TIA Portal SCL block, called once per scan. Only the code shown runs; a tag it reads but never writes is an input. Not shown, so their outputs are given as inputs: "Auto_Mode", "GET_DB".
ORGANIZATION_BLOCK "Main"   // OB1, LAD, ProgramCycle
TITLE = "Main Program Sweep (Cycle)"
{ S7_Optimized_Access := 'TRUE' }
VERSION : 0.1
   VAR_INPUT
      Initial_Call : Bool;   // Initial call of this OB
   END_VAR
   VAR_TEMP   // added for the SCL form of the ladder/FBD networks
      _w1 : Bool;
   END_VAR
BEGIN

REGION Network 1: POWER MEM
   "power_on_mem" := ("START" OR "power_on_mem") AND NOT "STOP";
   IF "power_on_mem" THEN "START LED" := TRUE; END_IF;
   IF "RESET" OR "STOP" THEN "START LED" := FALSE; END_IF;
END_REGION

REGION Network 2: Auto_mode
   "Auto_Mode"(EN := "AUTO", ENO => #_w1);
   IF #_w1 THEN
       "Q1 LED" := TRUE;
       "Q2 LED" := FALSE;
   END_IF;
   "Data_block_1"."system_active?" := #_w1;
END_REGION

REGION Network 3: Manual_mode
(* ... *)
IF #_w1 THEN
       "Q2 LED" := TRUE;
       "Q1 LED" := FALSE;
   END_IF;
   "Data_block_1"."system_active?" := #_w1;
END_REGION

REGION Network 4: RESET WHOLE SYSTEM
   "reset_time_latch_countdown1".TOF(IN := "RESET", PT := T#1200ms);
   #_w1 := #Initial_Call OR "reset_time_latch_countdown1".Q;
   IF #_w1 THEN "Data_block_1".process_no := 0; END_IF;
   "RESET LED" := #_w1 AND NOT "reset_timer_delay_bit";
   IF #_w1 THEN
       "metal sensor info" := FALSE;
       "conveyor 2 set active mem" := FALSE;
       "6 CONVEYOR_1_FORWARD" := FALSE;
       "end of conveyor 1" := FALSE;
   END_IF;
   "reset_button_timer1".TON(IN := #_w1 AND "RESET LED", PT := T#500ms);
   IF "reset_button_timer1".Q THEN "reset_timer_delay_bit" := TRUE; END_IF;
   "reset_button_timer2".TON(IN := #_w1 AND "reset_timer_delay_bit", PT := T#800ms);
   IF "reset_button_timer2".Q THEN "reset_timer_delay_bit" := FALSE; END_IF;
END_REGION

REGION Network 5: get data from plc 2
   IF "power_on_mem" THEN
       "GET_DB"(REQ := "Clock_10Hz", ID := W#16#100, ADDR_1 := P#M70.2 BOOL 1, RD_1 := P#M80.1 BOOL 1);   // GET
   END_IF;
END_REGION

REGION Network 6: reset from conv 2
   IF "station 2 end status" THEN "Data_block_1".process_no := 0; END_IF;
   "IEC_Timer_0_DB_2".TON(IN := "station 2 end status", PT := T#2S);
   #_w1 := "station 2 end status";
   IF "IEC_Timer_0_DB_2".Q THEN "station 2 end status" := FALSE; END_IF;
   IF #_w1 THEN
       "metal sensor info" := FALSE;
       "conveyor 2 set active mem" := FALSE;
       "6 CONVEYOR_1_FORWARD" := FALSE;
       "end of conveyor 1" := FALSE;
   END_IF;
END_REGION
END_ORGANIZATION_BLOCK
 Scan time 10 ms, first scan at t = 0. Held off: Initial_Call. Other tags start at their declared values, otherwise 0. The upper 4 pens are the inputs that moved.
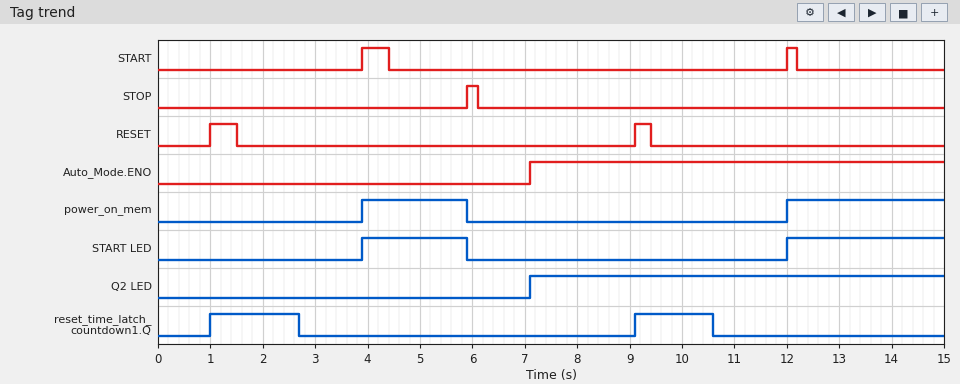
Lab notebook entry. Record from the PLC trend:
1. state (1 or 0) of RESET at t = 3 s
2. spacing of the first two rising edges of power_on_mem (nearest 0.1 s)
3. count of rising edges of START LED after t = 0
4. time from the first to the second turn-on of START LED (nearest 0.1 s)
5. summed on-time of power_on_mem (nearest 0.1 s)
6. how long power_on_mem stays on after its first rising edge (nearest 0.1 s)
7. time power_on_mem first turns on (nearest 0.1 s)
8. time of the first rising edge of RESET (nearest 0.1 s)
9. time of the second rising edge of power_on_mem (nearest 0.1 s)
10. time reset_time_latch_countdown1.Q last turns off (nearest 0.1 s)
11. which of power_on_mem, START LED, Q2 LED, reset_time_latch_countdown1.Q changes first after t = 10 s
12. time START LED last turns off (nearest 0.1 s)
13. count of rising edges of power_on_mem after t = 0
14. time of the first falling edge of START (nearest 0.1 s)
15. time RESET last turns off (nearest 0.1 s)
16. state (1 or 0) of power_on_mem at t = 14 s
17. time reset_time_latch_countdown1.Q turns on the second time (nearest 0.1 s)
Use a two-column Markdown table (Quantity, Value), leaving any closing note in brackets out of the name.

| Quantity | Value |
|---|---|
| state (1 or 0) of RESET at t = 3 s | 0 |
| spacing of the first two rising edges of power_on_mem | 8.1 s |
| count of rising edges of START LED after t = 0 | 2 |
| time from the first to the second turn-on of START LED | 8.1 s |
| summed on-time of power_on_mem | 5.0 s |
| how long power_on_mem stays on after its first rising edge | 2.0 s |
| time power_on_mem first turns on | 3.9 s |
| time of the first rising edge of RESET | 1.0 s |
| time of the second rising edge of power_on_mem | 12.0 s |
| time reset_time_latch_countdown1.Q last turns off | 10.6 s |
| which of power_on_mem, START LED, Q2 LED, reset_time_latch_countdown1.Q changes first after t = 10 s | reset_time_latch_countdown1.Q |
| time START LED last turns off | 5.9 s |
| count of rising edges of power_on_mem after t = 0 | 2 |
| time of the first falling edge of START | 4.4 s |
| time RESET last turns off | 9.4 s |
| state (1 or 0) of power_on_mem at t = 14 s | 1 |
| time reset_time_latch_countdown1.Q turns on the second time | 9.1 s |
